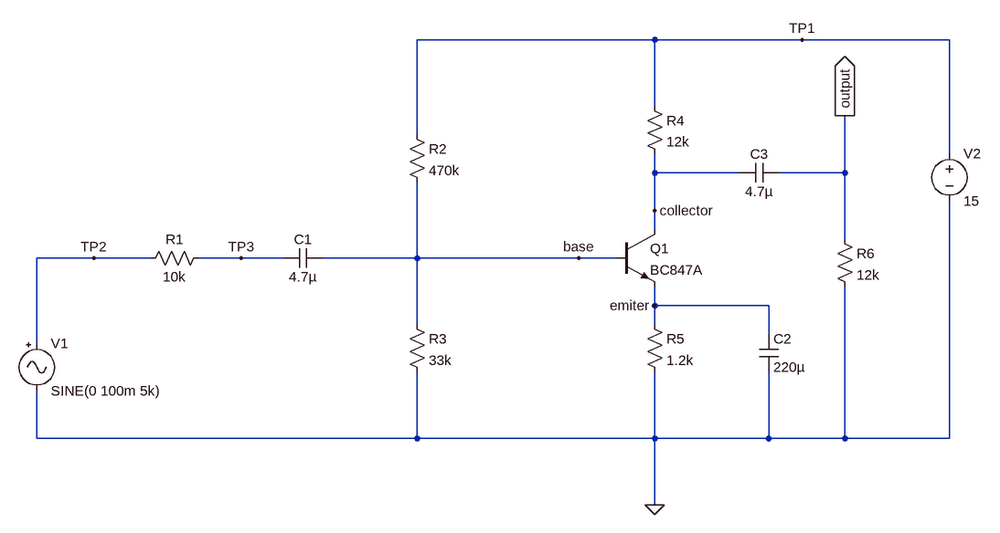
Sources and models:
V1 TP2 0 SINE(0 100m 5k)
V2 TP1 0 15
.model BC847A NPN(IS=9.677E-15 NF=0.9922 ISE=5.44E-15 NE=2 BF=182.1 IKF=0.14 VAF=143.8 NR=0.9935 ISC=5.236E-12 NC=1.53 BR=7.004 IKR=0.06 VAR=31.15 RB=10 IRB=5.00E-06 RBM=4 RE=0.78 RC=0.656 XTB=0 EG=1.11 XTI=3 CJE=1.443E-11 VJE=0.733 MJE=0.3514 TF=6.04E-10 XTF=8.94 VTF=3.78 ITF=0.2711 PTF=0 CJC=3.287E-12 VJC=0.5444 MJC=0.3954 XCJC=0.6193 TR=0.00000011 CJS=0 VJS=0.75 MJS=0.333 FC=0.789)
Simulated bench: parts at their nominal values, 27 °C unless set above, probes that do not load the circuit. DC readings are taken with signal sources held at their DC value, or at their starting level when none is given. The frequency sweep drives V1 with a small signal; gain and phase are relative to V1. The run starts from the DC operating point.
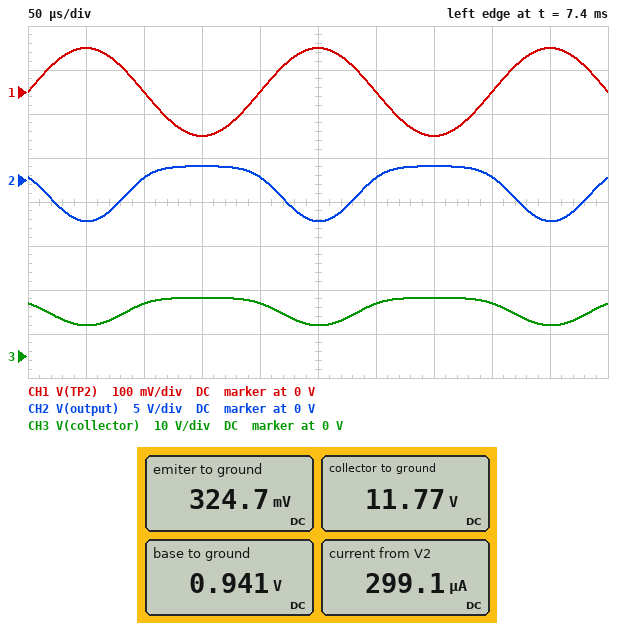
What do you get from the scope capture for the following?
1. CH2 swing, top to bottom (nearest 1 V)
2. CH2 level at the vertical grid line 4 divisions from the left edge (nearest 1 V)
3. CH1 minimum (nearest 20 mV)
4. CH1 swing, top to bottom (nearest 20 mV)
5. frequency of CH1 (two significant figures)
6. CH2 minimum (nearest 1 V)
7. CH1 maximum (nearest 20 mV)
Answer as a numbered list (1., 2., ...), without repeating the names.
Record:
1. 6 V
2. 0 V
3. -100 mV
4. 200 mV
5. 5.0 kHz
6. -5 V
7. 100 mV
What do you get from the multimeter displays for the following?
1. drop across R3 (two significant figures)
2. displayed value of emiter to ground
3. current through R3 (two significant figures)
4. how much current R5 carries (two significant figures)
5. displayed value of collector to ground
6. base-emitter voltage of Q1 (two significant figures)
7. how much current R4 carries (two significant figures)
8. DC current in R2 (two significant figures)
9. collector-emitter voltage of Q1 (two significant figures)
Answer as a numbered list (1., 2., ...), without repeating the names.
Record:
1. 940 mV
2. 324.7 mV
3. 29 µA
4. 270 µA
5. 11.77 V
6. 620 mV
7. 270 µA
8. 30 µA
9. 11 V
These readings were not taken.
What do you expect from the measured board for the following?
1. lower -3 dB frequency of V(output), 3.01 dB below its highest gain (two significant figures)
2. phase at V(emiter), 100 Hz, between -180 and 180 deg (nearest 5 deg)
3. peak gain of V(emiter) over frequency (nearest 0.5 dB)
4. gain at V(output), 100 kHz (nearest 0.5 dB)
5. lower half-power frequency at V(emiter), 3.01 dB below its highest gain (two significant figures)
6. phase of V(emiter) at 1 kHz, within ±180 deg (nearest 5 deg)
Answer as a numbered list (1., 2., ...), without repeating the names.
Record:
1. 7.0 Hz
2. -85 deg
3. -5.5 dB
4. 30.0 dB
5. 660 mHz
6. -90 deg
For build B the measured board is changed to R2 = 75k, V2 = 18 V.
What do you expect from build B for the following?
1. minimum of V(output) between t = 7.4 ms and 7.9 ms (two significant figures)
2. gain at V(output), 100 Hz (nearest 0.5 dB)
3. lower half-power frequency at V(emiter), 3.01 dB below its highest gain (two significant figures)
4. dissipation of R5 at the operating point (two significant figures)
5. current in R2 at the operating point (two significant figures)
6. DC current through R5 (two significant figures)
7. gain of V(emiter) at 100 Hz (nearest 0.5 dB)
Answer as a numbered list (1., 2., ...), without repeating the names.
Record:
1. -1.5 mV
2. -36.0 dB
3. 500 mHz
4. 2.6 mW
5. 210 µA
6. 1.5 mA
7. -62.5 dB
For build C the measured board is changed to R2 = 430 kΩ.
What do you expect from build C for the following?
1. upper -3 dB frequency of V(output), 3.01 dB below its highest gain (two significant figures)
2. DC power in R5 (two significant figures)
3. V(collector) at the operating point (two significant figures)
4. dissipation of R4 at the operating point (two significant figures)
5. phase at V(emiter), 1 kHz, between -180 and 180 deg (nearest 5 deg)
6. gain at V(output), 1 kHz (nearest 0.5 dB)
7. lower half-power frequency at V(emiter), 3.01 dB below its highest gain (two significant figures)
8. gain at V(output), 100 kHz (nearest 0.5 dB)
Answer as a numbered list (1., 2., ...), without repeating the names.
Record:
1. 280 kHz
2. 130 µW
3. 11 V
4. 1.3 mW
5. -90 deg
6. 31.5 dB
7. 670 mHz
8. 31.0 dB
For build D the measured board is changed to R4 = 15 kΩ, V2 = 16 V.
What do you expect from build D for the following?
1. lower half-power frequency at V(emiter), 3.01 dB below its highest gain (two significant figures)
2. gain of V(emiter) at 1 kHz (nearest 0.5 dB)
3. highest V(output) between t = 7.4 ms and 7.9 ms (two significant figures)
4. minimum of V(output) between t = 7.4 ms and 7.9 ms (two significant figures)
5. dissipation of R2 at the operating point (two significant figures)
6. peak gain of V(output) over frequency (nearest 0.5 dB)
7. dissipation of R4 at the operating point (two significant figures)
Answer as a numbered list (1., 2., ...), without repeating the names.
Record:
1. 670 mHz
2. -47.0 dB
3. 2.0 V
4. -5.5 V
5. 480 µW
6. 32.0 dB
7. 1.5 mW
